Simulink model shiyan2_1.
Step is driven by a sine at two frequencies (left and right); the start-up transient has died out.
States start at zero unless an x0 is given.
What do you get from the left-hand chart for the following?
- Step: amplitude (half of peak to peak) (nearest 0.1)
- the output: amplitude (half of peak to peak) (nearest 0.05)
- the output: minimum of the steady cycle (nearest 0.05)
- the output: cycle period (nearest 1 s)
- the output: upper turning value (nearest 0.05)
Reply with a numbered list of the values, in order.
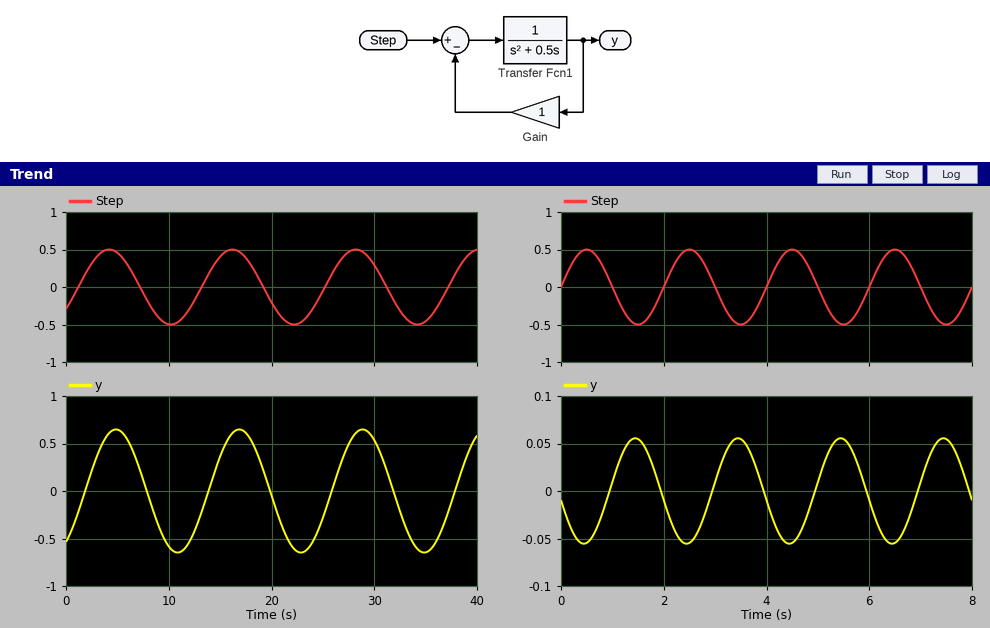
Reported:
1. 0.5
2. 0.65
3. -0.65
4. 12 s
5. 0.65
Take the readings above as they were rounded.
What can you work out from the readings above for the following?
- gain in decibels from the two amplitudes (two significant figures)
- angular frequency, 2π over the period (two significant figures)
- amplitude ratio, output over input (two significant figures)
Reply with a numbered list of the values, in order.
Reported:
1. 2.3 dB
2. 0.52 rad/s
3. 1.3
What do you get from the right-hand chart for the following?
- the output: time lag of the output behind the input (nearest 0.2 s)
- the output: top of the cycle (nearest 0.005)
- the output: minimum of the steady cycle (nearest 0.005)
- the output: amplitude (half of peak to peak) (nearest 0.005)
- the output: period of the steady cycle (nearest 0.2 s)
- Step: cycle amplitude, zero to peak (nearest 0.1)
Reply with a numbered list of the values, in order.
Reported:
1. 1.0 s
2. 0.055
3. -0.055
4. 0.055
5. 2.0 s
6. 0.5
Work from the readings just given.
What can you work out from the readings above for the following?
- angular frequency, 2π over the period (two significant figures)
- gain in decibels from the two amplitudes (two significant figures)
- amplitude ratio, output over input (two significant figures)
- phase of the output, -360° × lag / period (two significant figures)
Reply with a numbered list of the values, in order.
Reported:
1. 3.1 rad/s
2. -19 dB
3. 0.11
4. -180°
